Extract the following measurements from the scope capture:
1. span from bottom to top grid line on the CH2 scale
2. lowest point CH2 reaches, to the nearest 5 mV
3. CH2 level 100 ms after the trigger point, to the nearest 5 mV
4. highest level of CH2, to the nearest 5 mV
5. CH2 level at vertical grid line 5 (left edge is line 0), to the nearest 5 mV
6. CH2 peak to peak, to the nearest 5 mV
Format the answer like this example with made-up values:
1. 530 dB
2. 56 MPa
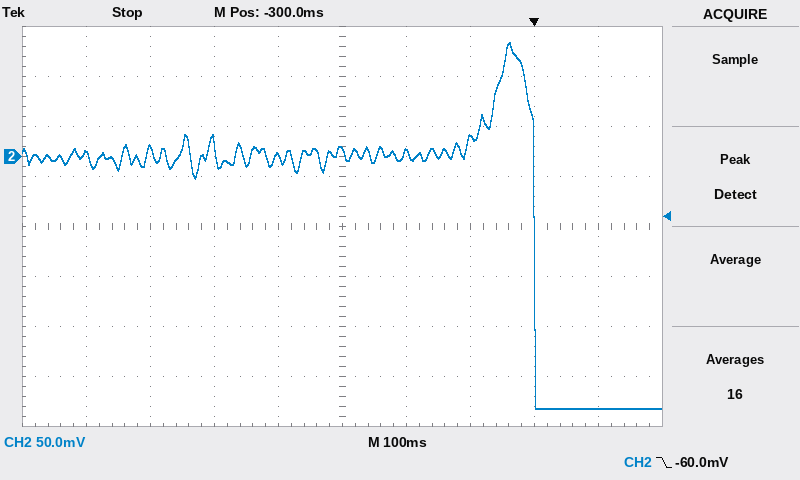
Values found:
1. 400 mV
2. -250 mV
3. -250 mV
4. 115 mV
5. 5 mV
6. 365 mV
